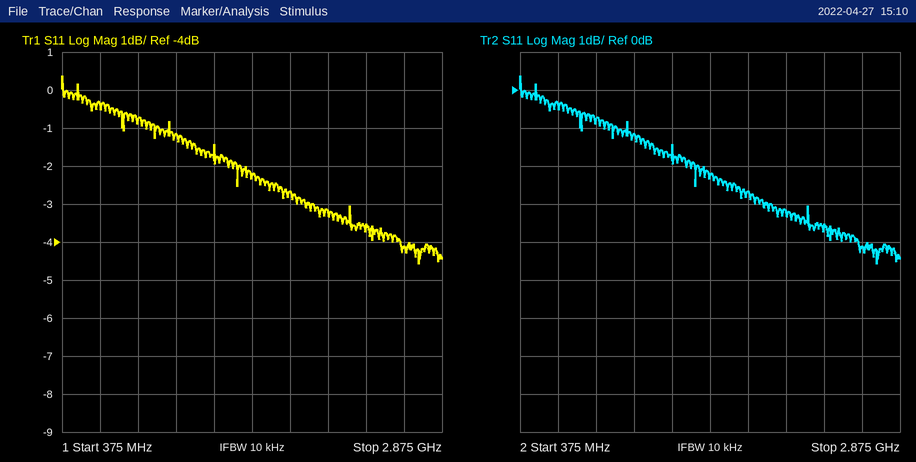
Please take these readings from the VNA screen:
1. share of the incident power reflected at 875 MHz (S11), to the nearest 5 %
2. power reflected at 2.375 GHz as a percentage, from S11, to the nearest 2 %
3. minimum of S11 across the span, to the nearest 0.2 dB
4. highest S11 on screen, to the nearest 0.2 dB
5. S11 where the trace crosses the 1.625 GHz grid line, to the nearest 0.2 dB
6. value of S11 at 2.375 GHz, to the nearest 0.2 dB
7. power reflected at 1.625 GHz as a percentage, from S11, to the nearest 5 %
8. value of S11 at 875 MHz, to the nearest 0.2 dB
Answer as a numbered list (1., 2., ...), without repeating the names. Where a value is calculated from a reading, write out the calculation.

1. 10^(-0.8/10) ≈ 83.2 %, so 85 % to the nearest 5 %
2. 10^(-3.6/10) ≈ 44 %
3. -4.6 dB
4. 0.4 dB
5. -2.2 dB
6. -3.6 dB
7. 10^(-2.2/10) ≈ 60 %
8. -0.8 dB
